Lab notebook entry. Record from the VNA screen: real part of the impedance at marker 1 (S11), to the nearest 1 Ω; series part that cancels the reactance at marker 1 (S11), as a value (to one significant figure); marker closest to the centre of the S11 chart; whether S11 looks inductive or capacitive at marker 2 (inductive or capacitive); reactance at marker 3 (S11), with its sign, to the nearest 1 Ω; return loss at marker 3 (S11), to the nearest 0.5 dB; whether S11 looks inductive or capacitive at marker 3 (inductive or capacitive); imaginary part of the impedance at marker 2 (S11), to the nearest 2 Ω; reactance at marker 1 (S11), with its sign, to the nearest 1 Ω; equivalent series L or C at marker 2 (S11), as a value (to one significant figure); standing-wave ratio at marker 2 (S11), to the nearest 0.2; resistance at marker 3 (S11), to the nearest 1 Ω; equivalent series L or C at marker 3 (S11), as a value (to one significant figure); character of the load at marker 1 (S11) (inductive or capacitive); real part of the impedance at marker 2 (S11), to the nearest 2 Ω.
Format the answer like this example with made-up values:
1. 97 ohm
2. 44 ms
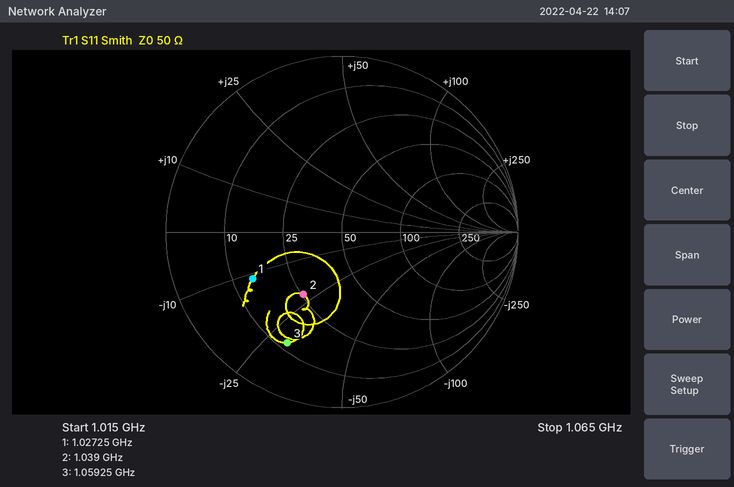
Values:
1. 14 Ω
2. 2 nH
3. marker 2
4. capacitive
5. -30 Ω
6. 3.0 dB
7. capacitive
8. -22 Ω
9. -11 Ω
10. 7 pF
11. 2.4
12. 12 Ω
13. 5 pF
14. capacitive
15. 26 Ω
